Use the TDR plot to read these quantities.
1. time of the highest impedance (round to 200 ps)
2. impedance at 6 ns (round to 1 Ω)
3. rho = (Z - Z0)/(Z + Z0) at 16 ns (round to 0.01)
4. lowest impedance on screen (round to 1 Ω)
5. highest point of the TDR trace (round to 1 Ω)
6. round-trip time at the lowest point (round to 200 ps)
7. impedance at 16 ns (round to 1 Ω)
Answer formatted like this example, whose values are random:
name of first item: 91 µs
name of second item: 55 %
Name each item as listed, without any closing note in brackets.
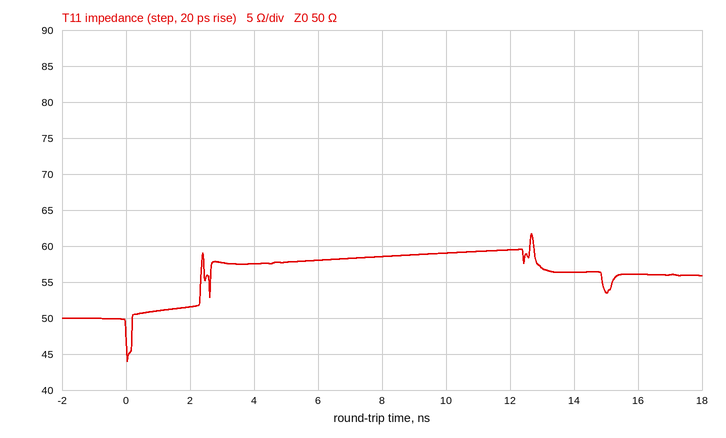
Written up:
time of the highest impedance: 12.6 ns
impedance at 6 ns: 58 Ω
rho = (Z - Z0)/(Z + Z0) at 16 ns: +0.06
lowest impedance on screen: 44 Ω
highest point of the TDR trace: 62 Ω
round-trip time at the lowest point: 0.0 ns
impedance at 16 ns: 56 Ω
